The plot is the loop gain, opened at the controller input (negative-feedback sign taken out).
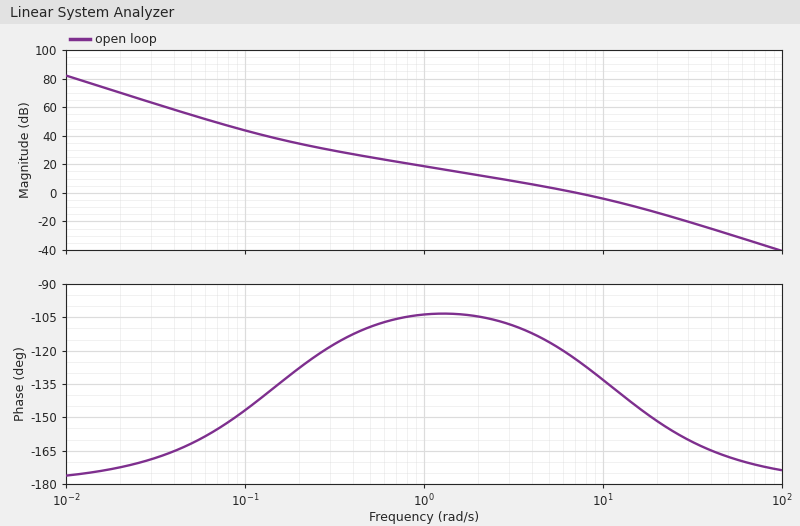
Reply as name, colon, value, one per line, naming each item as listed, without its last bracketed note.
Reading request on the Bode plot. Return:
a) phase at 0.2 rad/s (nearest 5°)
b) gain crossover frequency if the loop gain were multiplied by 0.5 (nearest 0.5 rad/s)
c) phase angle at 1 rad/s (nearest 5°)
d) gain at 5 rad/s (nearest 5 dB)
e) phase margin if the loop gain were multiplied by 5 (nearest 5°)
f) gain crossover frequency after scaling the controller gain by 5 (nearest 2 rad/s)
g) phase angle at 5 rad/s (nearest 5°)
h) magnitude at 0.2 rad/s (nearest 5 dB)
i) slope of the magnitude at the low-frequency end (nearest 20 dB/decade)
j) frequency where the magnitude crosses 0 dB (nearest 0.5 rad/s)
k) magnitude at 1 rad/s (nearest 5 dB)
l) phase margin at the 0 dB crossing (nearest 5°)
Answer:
phase at 0.2 rad/s: -130°
gain crossover frequency if the loop gain were multiplied by 0.5: 4.0 rad/s
phase angle at 1 rad/s: -105°
gain at 5 rad/s: 5 dB
phase margin if the loop gain were multiplied by 5: 30°
gain crossover frequency after scaling the controller gain by 5: 20 rad/s
phase angle at 5 rad/s: -115°
magnitude at 0.2 rad/s: 35 dB
slope of the magnitude at the low-frequency end: -40 dB/decade
frequency where the magnitude crosses 0 dB: 7.0 rad/s
magnitude at 1 rad/s: 20 dB
phase margin at the 0 dB crossing: 55°
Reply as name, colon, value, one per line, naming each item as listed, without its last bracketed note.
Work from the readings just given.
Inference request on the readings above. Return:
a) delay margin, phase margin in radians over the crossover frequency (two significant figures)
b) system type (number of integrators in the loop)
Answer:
delay margin, phase margin in radians over the crossover frequency: 0.14 s
system type: 2
